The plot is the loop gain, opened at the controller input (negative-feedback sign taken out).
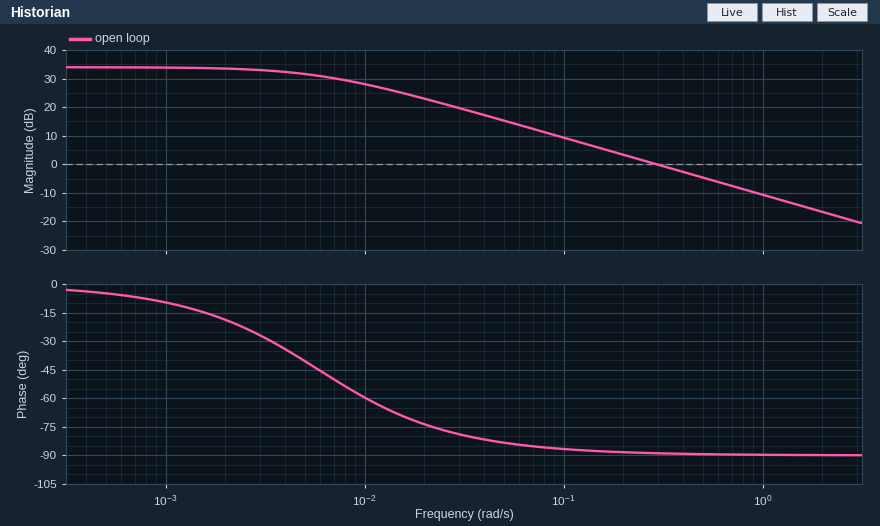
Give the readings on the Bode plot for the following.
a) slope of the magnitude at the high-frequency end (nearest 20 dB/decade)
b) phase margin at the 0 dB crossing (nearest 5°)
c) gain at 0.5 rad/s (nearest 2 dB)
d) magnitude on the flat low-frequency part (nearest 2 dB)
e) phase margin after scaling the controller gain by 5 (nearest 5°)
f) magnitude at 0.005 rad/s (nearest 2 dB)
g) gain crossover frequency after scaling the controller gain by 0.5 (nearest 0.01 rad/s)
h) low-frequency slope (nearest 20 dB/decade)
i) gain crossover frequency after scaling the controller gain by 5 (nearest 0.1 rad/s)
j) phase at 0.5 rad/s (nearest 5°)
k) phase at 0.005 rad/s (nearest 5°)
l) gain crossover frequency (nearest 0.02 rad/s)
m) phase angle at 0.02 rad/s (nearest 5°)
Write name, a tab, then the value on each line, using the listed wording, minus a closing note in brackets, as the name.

slope of the magnitude at the high-frequency end	-20 dB/decade
phase margin at the 0 dB crossing	90°
gain at 0.5 rad/s	-4 dB
magnitude on the flat low-frequency part	34 dB
phase margin after scaling the controller gain by 5	90°
magnitude at 0.005 rad/s	32 dB
gain crossover frequency after scaling the controller gain by 0.5	0.15 rad/s
low-frequency slope	0 dB/decade
gain crossover frequency after scaling the controller gain by 5	1.5 rad/s
phase at 0.5 rad/s	-90°
phase at 0.005 rad/s	-40°
gain crossover frequency	0.30 rad/s
phase angle at 0.02 rad/s	-75°
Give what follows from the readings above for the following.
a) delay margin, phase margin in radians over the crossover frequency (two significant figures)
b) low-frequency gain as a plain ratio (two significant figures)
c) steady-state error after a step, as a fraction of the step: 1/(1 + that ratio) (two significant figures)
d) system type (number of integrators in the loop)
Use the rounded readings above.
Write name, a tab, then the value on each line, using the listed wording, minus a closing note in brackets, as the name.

delay margin, phase margin in radians over the crossover frequency	5.2 s
low-frequency gain as a plain ratio	50
steady-state error after a step, as a fraction of the step: 1/(1 + that ratio)	0.020
system type	0
